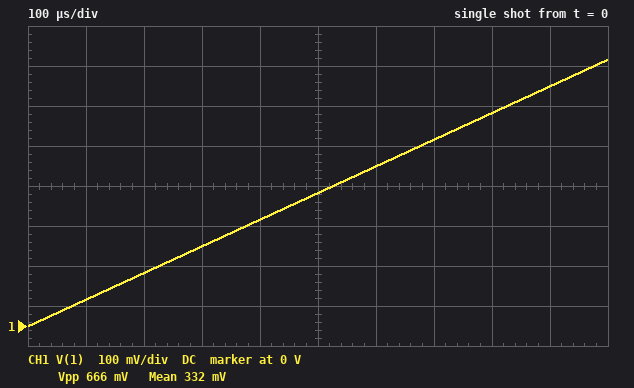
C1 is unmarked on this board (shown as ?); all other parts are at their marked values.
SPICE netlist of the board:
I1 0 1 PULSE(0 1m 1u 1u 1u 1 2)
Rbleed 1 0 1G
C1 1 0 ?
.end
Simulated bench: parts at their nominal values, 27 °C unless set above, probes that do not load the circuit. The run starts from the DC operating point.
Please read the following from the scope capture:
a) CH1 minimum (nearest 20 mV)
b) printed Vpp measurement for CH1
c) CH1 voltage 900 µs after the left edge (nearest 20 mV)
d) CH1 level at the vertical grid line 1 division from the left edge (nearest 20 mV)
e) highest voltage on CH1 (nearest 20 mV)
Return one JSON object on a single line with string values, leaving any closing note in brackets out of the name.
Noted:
{"CH1 minimum": "0 V", "printed Vpp measurement for CH1": "666 mV", "CH1 voltage 900 µs after the left edge": "600 mV", "CH1 level at the vertical grid line 1 division from the left edge": "60 mV", "highest voltage on CH1": "660 mV"}
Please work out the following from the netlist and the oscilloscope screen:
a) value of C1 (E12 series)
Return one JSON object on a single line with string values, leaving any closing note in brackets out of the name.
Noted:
{"value of C1": "1.5 µF"}
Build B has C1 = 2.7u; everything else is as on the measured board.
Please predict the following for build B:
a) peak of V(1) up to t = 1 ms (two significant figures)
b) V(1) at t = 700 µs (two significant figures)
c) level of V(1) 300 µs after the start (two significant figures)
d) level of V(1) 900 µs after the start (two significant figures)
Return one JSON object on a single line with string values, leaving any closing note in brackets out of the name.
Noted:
{"peak of V(1) up to t = 1 ms": "370 mV", "V(1) at t = 700 µs": "260 mV", "level of V(1) 300 µs after the start": "110 mV", "level of V(1) 900 µs after the start": "330 mV"}
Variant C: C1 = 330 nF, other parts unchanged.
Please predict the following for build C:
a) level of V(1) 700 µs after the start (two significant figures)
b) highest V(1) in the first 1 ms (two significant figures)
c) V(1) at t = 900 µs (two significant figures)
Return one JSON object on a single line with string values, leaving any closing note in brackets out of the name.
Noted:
{"level of V(1) 700 µs after the start": "2.1 V", "highest V(1) in the first 1 ms": "3.0 V", "V(1) at t = 900 µs": "2.7 V"}
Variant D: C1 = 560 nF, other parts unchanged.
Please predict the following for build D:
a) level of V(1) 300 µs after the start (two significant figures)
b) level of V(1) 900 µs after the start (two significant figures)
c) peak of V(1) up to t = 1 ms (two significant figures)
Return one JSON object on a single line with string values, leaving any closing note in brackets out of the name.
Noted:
{"level of V(1) 300 µs after the start": "530 mV", "level of V(1) 900 µs after the start": "1.6 V", "peak of V(1) up to t = 1 ms": "1.8 V"}
